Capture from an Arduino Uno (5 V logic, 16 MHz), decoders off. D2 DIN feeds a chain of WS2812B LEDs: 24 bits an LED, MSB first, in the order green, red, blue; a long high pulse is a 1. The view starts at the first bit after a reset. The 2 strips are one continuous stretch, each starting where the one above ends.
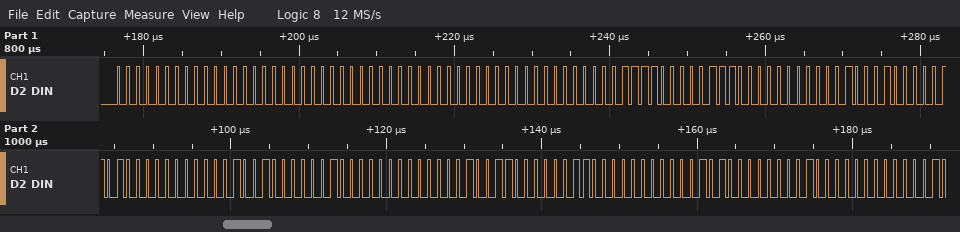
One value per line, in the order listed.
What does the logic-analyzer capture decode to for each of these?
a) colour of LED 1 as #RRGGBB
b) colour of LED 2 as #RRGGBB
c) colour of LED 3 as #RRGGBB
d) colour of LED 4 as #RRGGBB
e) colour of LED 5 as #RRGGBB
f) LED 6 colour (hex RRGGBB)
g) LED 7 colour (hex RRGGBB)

#000000
#000000
#070F00
#051100
#041200
#031300
#021400
